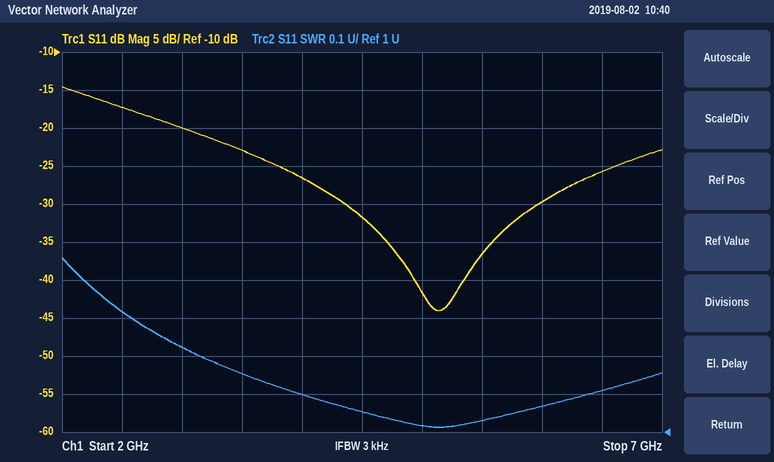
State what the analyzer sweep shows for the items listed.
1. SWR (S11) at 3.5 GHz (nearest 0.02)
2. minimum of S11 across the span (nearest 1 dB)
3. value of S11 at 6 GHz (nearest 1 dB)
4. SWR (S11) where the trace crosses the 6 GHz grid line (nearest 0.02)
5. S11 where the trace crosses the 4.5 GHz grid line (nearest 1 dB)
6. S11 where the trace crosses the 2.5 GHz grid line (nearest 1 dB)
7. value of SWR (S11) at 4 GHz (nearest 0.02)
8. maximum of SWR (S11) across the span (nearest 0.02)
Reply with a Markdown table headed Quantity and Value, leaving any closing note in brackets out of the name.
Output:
| Quantity | Value |
|---|---|
| SWR (S11) at 3.5 GHz | 1.16 |
| minimum of S11 across the span | -44 dB |
| value of S11 at 6 GHz | -30 dB |
| SWR (S11) where the trace crosses the 6 GHz grid line | 1.06 |
| S11 where the trace crosses the 4.5 GHz grid line | -32 dB |
| S11 where the trace crosses the 2.5 GHz grid line | -17 dB |
| value of SWR (S11) at 4 GHz | 1.10 |
| maximum of SWR (S11) across the span | 1.46 |
